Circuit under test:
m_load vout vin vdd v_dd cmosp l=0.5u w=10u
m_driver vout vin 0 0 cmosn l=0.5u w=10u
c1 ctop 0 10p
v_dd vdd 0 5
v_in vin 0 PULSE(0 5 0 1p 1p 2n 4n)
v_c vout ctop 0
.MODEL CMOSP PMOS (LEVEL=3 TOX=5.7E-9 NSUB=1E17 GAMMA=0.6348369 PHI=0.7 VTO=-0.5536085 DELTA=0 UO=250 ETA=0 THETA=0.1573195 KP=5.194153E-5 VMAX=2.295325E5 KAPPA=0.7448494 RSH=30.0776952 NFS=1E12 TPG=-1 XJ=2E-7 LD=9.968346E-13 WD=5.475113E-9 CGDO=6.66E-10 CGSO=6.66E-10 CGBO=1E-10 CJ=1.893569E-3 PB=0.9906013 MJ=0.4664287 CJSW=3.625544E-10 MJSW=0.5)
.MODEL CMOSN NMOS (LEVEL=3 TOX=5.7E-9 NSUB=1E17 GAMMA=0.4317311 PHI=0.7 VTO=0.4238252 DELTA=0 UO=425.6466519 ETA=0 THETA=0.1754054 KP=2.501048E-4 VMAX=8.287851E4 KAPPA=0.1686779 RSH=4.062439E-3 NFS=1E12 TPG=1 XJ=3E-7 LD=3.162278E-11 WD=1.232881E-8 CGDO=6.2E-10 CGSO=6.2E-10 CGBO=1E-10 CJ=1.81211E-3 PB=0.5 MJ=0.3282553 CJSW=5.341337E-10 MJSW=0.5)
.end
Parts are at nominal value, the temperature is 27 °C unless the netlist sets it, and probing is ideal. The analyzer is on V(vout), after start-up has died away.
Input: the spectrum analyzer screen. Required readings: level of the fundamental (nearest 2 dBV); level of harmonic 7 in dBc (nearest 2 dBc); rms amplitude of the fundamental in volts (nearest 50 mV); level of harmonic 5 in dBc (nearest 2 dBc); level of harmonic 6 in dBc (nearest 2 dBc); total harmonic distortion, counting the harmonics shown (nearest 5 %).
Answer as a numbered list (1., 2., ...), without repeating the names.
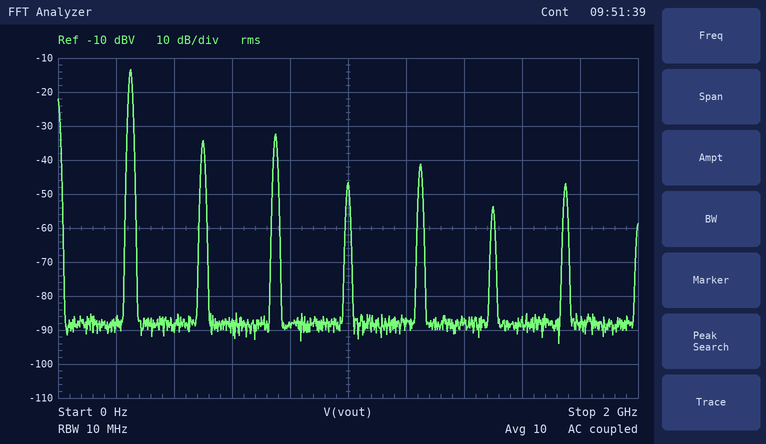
1. -14 dBV
2. -34 dBc
3. 200 mV
4. -28 dBc
5. -40 dBc
6. 15 %
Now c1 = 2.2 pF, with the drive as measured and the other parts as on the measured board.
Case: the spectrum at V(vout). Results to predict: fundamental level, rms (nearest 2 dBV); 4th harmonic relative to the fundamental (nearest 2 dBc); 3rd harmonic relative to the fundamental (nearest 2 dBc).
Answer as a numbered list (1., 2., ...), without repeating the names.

1. 0 dBV
2. -28 dBc
3. -16 dBc
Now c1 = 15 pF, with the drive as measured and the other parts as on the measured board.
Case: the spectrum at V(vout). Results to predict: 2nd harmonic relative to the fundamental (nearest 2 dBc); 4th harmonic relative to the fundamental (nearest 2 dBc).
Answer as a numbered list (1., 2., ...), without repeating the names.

1. -24 dBc
2. -36 dBc
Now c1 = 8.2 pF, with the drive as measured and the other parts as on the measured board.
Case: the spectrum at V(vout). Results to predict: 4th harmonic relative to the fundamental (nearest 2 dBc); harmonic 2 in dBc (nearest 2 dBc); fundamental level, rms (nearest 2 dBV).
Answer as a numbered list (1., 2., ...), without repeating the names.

1. -32 dBc
2. -20 dBc
3. -12 dBV
